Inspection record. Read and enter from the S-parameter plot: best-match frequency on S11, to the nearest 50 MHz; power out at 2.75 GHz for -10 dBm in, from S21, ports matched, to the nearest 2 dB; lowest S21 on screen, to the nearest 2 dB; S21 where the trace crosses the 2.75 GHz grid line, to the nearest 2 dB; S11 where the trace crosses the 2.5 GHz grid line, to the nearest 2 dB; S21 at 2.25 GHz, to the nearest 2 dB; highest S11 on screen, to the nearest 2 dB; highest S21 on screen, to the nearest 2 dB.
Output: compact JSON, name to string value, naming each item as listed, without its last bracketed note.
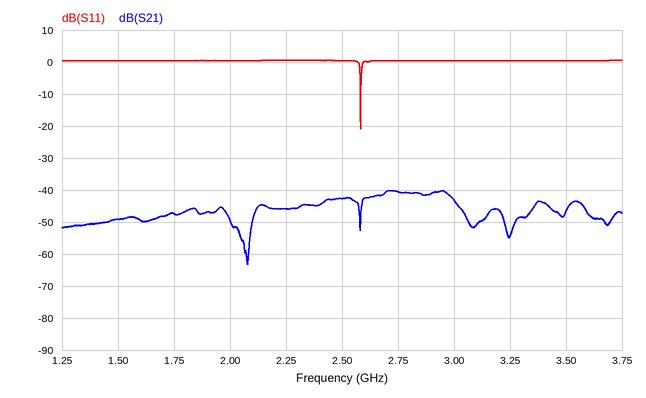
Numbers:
{"best-match frequency on S11, to the nearest 50 MHz": "2.60 GHz", "power out at 2.75 GHz for -10 dBm in, from S21, ports matched, to the nearest 2 dB": "-50 dBm", "lowest S21 on screen, to the nearest 2 dB": "-64 dB", "S21 where the trace crosses the 2.75 GHz grid line, to the nearest 2 dB": "-40 dB", "S11 where the trace crosses the 2.5 GHz grid line, to the nearest 2 dB": "0 dB", "S21 at 2.25 GHz, to the nearest 2 dB": "-46 dB", "highest S11 on screen, to the nearest 2 dB": "0 dB", "highest S21 on screen, to the nearest 2 dB": "-40 dB"}
